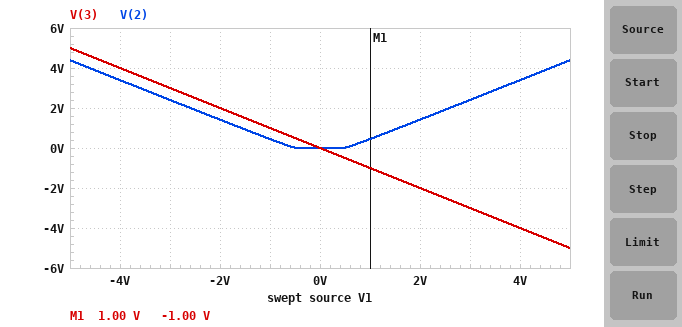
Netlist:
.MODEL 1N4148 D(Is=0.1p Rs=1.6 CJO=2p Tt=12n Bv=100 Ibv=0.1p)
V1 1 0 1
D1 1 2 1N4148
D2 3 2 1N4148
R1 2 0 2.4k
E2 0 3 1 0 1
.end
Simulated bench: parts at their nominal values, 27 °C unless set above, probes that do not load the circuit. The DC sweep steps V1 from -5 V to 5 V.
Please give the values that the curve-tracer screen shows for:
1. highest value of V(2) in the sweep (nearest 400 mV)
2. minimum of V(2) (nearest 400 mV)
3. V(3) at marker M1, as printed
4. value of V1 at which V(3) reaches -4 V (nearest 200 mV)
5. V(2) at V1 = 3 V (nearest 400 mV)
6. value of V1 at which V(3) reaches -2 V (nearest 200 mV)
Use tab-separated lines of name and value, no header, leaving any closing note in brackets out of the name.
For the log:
highest value of V(2) in the sweep	4.4 V
minimum of V(2)	0 V
V(3) at marker M1, as printed	-1.00 V
value of V1 at which V(3) reaches -4 V	4.0 V
V(2) at V1 = 3 V	2.4 V
value of V1 at which V(3) reaches -2 V	2.0 V
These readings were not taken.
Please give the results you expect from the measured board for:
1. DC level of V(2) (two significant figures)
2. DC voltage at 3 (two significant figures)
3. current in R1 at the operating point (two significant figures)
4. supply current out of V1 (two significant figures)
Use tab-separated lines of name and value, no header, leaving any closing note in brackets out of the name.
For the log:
DC level of V(2)	450 mV
DC voltage at 3	-1.0 V
current in R1 at the operating point	190 µA
supply current out of V1	190 µA
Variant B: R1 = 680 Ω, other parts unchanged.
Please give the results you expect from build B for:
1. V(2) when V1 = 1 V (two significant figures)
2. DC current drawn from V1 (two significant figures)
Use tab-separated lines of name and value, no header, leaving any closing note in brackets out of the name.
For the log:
V(2) when V1 = 1 V	420 mV
DC current drawn from V1	610 µA
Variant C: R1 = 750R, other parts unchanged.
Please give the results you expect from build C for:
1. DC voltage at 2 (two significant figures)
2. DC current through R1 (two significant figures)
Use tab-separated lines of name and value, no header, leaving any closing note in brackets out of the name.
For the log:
DC voltage at 2	420 mV
DC current through R1	560 µA
